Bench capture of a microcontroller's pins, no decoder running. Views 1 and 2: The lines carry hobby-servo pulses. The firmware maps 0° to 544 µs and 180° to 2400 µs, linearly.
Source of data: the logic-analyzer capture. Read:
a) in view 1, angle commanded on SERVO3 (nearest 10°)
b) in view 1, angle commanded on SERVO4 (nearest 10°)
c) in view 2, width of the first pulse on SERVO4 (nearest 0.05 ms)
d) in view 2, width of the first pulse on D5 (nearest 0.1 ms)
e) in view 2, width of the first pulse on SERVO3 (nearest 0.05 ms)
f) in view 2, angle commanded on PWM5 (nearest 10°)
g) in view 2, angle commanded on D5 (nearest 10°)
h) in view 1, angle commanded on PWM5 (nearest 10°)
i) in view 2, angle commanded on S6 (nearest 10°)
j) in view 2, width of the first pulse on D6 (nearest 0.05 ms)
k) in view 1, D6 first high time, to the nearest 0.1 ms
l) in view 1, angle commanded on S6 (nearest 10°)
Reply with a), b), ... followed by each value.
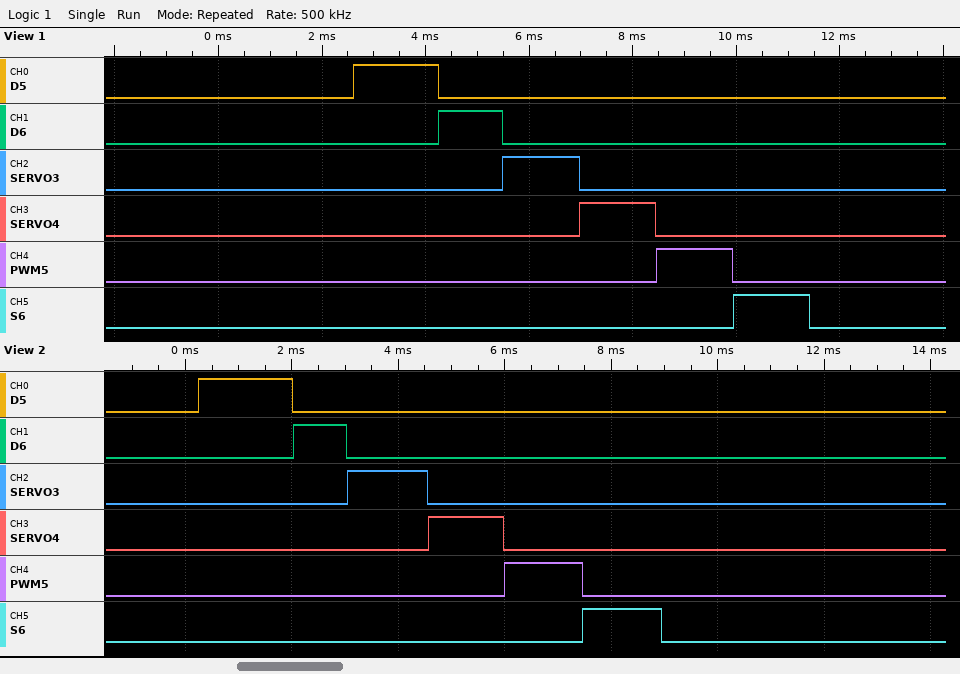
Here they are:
a) 90°
b) 90°
c) 1.40 ms
d) 1.8 ms
e) 1.50 ms
f) 90°
g) 120°
h) 90°
i) 90°
j) 1.00 ms
k) 1.2 ms
l) 90°
